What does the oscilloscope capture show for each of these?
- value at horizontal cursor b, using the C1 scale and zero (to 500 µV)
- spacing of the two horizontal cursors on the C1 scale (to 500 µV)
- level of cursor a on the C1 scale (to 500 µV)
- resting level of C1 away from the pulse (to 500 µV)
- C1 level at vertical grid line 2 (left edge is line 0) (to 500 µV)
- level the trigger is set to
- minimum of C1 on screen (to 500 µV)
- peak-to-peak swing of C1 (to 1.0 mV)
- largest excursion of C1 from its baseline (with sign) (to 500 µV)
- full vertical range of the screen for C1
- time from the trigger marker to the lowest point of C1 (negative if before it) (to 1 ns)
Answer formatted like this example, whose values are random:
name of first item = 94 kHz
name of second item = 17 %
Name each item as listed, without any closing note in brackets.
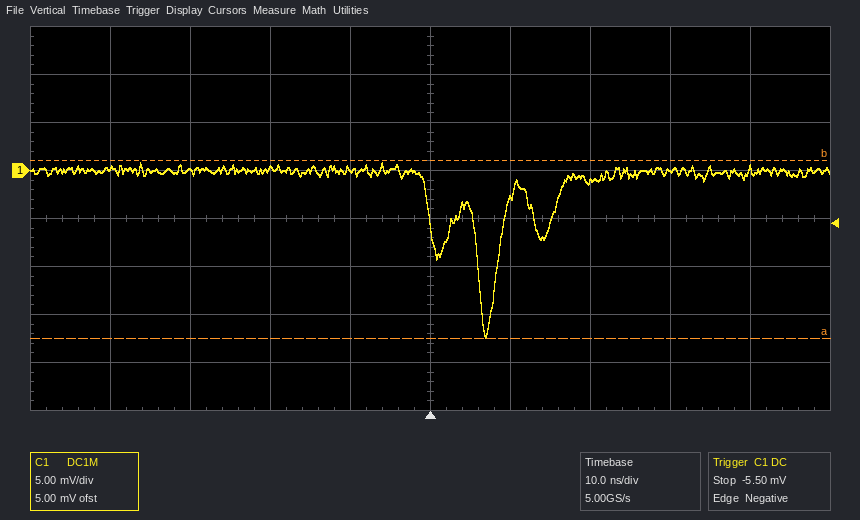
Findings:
value at horizontal cursor b, using the C1 scale and zero = 1.0 mV
spacing of the two horizontal cursors on the C1 scale = 18.5 mV
level of cursor a on the C1 scale = -17.5 mV
resting level of C1 away from the pulse = 0.0 mV
C1 level at vertical grid line 2 (left edge is line 0) = 0.0 mV
level the trigger is set to = -5.50 mV
minimum of C1 on screen = -17.5 mV
peak-to-peak swing of C1 = 18.0 mV
largest excursion of C1 from its baseline (with sign) = -17.5 mV
full vertical range of the screen for C1 = 40 mV
time from the trigger marker to the lowest point of C1 (negative if before it) = +7 ns
